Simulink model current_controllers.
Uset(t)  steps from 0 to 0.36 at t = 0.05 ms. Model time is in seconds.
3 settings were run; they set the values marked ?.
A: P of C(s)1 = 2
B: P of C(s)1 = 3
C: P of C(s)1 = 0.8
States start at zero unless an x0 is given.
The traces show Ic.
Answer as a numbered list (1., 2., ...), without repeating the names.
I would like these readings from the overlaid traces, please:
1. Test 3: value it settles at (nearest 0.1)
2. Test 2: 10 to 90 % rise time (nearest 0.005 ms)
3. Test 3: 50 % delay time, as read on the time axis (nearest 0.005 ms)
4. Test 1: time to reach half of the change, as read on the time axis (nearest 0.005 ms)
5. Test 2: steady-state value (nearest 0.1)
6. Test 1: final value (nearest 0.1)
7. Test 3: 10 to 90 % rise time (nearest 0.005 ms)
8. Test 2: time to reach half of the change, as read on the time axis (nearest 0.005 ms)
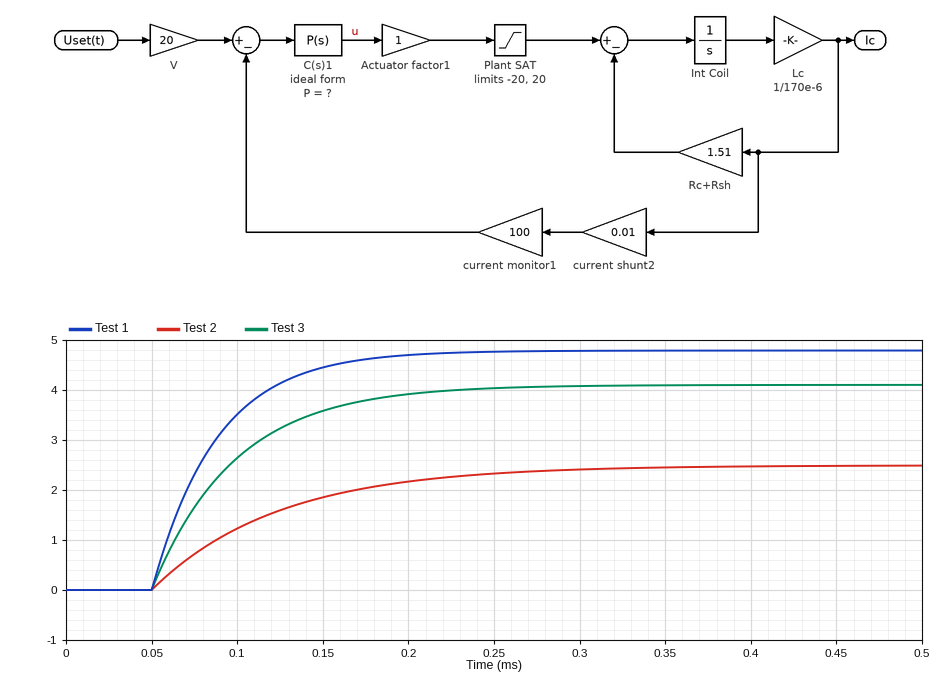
1. 4.1
2. 0.160 ms
3. 0.085 ms
4. 0.075 ms
5. 2.5
6. 4.8
7. 0.105 ms
8. 0.100 ms
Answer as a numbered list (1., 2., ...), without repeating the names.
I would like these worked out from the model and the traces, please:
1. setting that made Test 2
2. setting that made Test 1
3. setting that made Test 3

1. C
2. B
3. A
